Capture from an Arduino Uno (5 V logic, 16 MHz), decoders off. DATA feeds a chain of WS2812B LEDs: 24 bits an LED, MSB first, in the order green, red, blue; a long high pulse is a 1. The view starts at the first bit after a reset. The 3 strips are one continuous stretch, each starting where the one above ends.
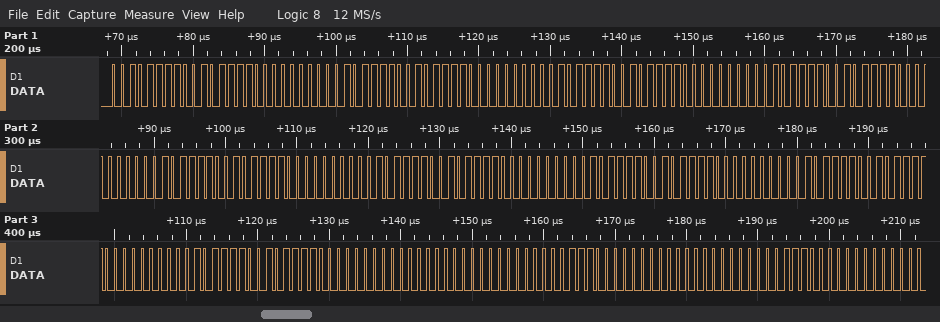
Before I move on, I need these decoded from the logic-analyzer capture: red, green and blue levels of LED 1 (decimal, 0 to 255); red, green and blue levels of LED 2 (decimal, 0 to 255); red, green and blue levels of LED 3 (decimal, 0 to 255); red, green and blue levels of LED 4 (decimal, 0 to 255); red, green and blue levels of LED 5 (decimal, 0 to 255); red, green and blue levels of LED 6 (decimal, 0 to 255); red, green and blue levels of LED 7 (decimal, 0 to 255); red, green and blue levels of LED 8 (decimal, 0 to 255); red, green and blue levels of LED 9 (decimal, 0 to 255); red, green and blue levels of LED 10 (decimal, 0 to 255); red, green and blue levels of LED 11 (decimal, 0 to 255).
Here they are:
47, 47, 0
47, 47, 0
47, 47, 0
47, 47, 0
47, 47, 0
47, 47, 0
47, 47, 0
47, 47, 0
47, 47, 0
0, 0, 14
0, 0, 14
